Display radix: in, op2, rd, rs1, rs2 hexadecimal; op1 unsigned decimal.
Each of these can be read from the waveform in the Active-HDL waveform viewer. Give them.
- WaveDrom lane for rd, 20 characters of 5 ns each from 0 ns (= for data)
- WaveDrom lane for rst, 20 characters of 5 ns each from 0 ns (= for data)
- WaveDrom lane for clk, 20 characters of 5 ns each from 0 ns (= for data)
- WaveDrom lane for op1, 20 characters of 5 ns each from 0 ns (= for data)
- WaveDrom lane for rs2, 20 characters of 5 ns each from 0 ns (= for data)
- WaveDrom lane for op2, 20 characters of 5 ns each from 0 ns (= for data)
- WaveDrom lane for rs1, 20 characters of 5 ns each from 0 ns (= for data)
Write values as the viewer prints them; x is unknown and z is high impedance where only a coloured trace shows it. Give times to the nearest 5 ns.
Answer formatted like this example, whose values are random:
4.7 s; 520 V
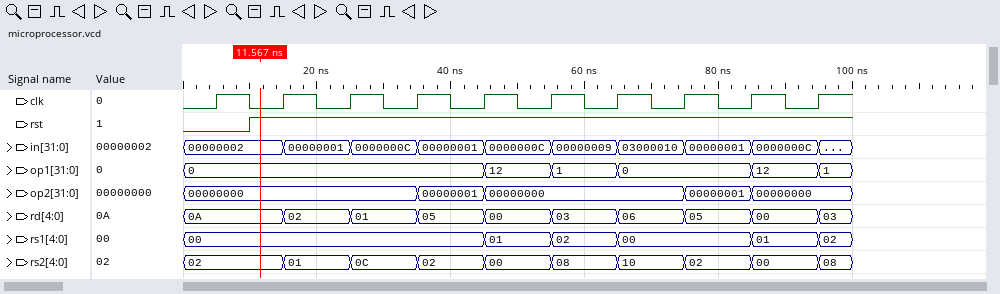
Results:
{name: 'rd', wave: '=..=.=.=.=.=.=.=.=.=', data: '0A 02 01 05 00 03 06 05 00 03'}; {name: 'rst', wave: '0.1.................'}; {name: 'clk', wave: '01010101010101010101'}; {name: 'op1', wave: '=........=.=.=...=.=', data: '0 12 1 0 12 1'}; {name: 'rs2', wave: '=..=.=.=.=.=.=.=.=.=', data: '02 01 0C 02 00 08 10 02 00 08'}; {name: 'op2', wave: '=......=.=.....=.=..', data: '00000000 00000001 00000000 00000001 00000000'}; {name: 'rs1', wave: '=........=.=.=...=.=', data: '00 01 02 00 01 02'}
